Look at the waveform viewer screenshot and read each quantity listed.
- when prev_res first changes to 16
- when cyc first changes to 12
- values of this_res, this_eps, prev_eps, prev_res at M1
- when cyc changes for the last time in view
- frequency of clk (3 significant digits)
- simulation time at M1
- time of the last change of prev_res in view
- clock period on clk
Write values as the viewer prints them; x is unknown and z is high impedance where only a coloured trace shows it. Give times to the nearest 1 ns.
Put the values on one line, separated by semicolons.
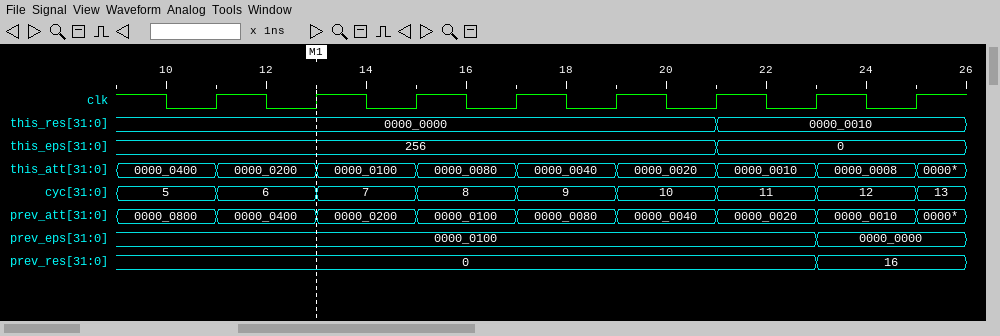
23 ns; 23 ns; this_res=0000_0000, this_eps=256, prev_eps=0000_0100, prev_res=0; 25 ns; 500 MHz; 13 ns; 23 ns; 2 ns
